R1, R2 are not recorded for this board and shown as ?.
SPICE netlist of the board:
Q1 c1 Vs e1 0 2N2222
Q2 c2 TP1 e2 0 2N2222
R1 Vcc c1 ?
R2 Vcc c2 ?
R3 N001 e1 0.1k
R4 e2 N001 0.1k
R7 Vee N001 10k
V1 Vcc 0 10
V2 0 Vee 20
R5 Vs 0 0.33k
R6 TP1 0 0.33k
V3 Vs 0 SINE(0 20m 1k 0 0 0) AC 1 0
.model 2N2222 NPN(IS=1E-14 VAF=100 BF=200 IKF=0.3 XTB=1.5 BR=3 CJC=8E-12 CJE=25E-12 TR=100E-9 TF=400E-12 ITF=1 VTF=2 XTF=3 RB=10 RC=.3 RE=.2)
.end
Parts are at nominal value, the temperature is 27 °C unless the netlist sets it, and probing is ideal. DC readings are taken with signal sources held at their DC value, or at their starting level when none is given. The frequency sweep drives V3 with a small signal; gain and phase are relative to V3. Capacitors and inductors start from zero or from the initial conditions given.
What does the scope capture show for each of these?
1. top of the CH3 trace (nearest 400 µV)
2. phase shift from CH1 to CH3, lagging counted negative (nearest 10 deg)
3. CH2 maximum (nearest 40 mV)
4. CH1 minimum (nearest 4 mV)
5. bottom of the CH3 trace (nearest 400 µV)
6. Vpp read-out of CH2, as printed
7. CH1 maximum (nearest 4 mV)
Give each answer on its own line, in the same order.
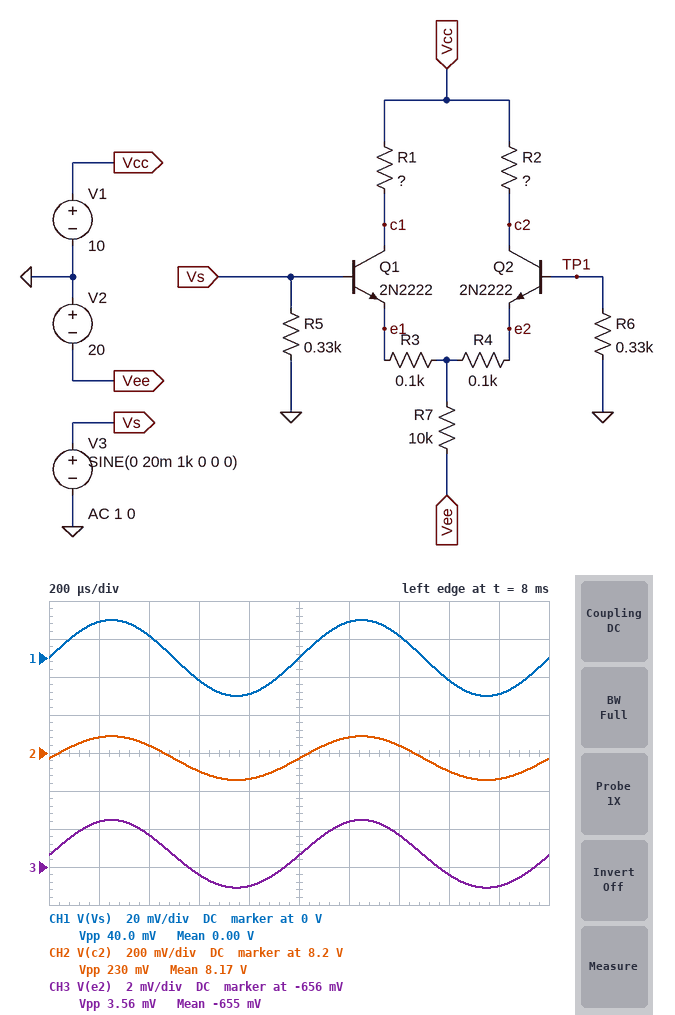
-653.6 mV
0 deg
8.28 V
-20 mV
-657.2 mV
230 mV
20 mV
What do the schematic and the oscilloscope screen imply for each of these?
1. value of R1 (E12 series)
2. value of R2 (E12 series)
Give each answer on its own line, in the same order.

15 kΩ
1.8 kΩ
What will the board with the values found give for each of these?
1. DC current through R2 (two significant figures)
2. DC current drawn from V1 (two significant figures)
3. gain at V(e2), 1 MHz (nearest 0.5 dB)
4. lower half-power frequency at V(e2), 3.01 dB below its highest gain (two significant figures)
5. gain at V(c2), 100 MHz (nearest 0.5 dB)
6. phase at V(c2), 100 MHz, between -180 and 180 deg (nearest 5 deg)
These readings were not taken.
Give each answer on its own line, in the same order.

1.0 mA
1.7 mA
-18.5 dB
8.2 MHz
-7.5 dB
-55 deg
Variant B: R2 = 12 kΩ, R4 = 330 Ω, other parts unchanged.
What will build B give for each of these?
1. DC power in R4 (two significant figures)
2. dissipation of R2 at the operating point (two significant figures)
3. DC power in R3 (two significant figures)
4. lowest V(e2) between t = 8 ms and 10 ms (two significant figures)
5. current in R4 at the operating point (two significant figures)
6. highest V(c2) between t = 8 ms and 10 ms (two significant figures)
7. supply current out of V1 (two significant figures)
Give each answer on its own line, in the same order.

110 µW
3.8 mW
180 µW
-640 mV
570 µA
3.7 V
1.3 mA
